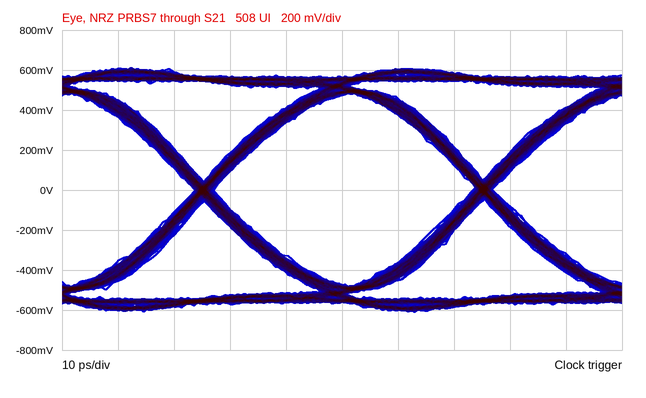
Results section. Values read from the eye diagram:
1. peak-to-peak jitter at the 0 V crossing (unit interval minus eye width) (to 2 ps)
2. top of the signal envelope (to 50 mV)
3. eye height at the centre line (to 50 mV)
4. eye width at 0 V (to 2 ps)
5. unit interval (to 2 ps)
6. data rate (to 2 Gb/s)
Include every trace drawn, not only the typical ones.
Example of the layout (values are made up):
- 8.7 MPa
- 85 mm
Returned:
- 4 ps
- 600 mV
- 950 mV
- 46 ps
- 50 ps
- 20 Gb/s
